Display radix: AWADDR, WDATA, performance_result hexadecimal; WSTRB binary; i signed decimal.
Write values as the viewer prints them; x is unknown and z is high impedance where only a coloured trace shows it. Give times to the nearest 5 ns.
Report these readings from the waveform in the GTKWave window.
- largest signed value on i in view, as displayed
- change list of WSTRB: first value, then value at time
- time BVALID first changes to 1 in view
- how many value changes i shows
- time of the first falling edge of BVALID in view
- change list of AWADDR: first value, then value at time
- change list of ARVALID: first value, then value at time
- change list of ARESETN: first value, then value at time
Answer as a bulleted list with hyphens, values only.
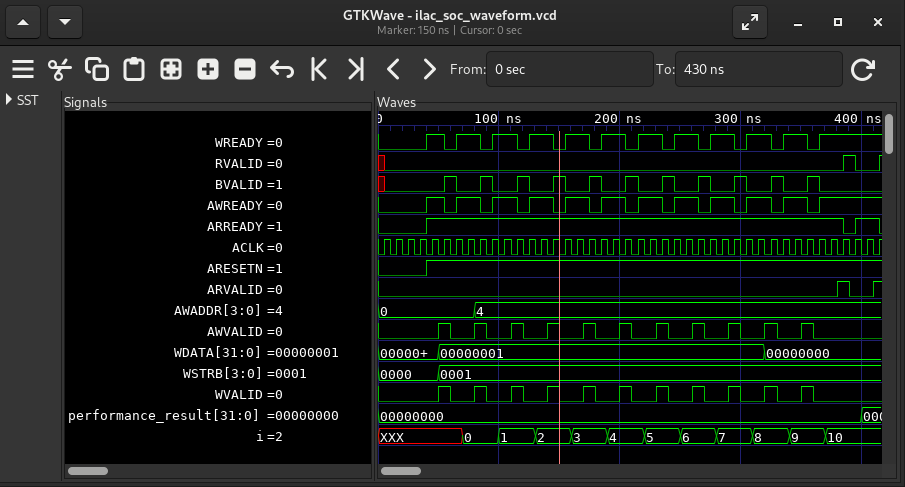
- 10
- 0000, 0001 at 50 ns
- 55 ns
- 11
- 65 ns
- 0, 4 at 80 ns
- 0, 1 at 380 ns, 0 at 390 ns, 1 at 410 ns
- 0, 1 at 40 ns
